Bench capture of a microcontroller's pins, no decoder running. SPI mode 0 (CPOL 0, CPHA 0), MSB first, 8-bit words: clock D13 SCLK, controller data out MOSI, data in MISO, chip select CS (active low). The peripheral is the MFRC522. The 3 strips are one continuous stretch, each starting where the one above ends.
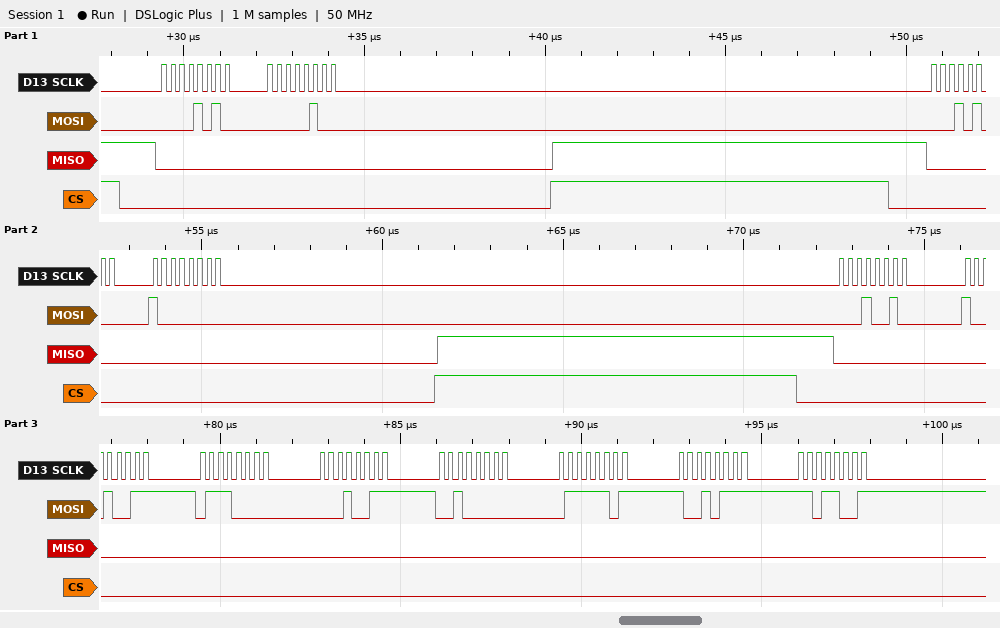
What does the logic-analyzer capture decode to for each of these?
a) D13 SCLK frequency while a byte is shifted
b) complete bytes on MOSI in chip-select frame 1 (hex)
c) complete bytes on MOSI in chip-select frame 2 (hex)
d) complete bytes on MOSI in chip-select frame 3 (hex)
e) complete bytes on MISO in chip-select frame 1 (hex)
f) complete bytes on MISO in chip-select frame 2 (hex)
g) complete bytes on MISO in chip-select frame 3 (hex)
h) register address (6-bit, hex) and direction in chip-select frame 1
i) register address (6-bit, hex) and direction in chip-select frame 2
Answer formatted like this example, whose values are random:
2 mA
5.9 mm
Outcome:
4 MHz
0A 04
14 80
12 93 70 13 20 7D 97 D9
00 00
00 00
00 00 00 00 00 00 00 00
0x05 write
0x0A write
